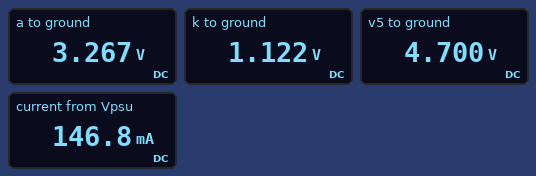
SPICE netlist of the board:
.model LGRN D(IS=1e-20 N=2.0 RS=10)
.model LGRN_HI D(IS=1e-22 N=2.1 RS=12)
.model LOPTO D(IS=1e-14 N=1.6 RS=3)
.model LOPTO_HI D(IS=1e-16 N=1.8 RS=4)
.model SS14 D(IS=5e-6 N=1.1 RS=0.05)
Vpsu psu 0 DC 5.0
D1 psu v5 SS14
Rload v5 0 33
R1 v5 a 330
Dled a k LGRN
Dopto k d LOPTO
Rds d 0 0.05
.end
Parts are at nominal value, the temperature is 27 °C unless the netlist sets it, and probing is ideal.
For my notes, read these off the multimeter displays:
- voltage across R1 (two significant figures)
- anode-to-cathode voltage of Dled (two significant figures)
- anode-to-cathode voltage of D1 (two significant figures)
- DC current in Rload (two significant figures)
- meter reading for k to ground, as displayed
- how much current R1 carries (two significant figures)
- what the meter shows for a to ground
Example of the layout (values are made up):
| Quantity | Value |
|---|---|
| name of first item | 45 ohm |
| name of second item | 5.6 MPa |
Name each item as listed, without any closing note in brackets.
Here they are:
| Quantity | Value |
|---|---|
| voltage across R1 | 1.4 V |
| anode-to-cathode voltage of Dled | 2.1 V |
| anode-to-cathode voltage of D1 | 300 mV |
| DC current in Rload | 140 mA |
| meter reading for k to ground, as displayed | 1.122 V |
| how much current R1 carries | 4.3 mA |
| what the meter shows for a to ground | 3.267 V |
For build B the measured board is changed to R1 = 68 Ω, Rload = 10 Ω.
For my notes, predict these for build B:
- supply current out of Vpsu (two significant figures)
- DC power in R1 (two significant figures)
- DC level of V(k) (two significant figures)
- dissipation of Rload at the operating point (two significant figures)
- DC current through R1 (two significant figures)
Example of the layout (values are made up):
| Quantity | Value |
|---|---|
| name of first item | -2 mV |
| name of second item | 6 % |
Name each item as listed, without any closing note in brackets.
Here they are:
| Quantity | Value |
|---|---|
| supply current out of Vpsu | 480 mA |
| DC power in R1 | 18 mW |
| DC level of V(k) | 1.2 V |
| dissipation of Rload at the operating point | 2.2 W |
| DC current through R1 | 16 mA |
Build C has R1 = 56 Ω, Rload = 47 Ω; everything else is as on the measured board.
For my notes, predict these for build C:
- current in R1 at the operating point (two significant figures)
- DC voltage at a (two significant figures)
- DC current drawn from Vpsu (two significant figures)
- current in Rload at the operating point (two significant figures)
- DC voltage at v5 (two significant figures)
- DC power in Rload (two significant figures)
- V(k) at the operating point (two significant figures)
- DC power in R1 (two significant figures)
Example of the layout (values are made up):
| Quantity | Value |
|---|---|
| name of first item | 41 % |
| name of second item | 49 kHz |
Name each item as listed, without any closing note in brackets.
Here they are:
| Quantity | Value |
|---|---|
| current in R1 at the operating point | 20 mA |
| DC voltage at a | 3.6 V |
| DC current drawn from Vpsu | 120 mA |
| current in Rload at the operating point | 100 mA |
| DC voltage at v5 | 4.7 V |
| DC power in Rload | 470 mW |
| V(k) at the operating point | 1.2 V |
| DC power in R1 | 22 mW |
